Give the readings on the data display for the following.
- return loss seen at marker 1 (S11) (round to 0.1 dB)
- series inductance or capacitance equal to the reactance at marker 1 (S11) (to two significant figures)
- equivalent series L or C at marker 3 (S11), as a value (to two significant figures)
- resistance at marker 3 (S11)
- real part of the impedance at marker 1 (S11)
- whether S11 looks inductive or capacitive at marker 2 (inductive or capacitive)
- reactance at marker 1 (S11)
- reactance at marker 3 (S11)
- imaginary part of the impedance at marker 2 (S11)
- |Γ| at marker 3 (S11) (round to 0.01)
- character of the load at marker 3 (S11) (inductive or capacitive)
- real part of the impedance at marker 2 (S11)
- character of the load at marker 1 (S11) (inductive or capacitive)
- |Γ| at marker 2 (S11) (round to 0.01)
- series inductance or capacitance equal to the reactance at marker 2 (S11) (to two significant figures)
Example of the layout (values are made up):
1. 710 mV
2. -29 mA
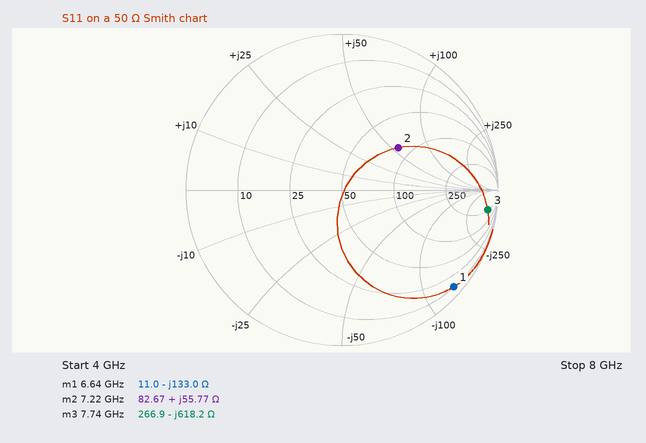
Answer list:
1. 0.5 dB
2. 180 fF
3. 33 fF
4. 266.9 Ω
5. 11.0 Ω
6. inductive
7. -133.0 Ω
8. -618.2 Ω
9. +55.77 Ω
10. 0.94
11. capacitive
12. 82.67 Ω
13. capacitive
14. 0.45
15. 1.2 nH
